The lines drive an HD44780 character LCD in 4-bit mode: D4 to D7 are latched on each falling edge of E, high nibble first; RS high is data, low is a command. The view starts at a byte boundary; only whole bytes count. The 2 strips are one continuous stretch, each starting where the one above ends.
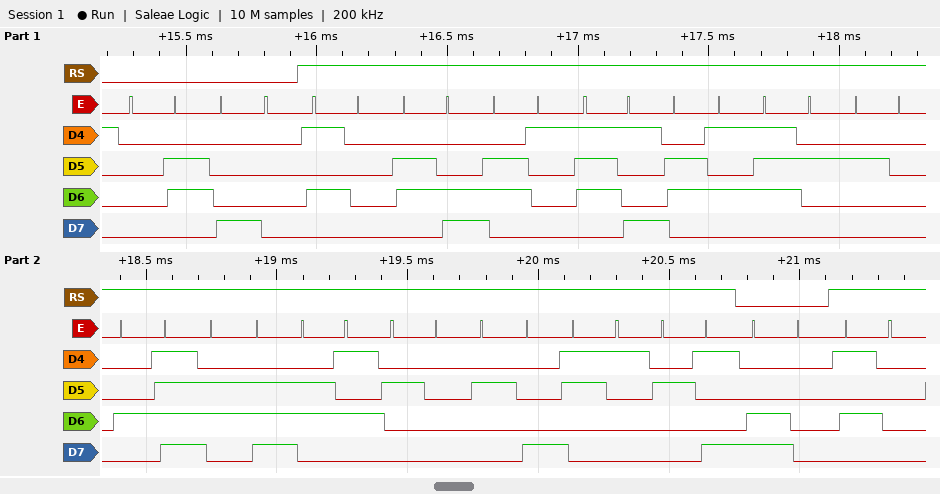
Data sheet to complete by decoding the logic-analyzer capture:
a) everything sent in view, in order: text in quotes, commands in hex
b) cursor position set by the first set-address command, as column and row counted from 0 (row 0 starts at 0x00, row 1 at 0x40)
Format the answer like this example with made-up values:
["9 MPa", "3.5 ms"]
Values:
["0x06 0x80 \"Player One (1)\" 0xC0 \"P\"", "column 0, row 0"]
